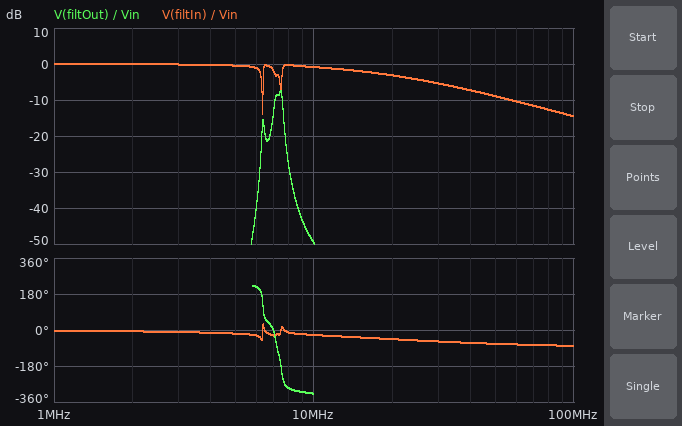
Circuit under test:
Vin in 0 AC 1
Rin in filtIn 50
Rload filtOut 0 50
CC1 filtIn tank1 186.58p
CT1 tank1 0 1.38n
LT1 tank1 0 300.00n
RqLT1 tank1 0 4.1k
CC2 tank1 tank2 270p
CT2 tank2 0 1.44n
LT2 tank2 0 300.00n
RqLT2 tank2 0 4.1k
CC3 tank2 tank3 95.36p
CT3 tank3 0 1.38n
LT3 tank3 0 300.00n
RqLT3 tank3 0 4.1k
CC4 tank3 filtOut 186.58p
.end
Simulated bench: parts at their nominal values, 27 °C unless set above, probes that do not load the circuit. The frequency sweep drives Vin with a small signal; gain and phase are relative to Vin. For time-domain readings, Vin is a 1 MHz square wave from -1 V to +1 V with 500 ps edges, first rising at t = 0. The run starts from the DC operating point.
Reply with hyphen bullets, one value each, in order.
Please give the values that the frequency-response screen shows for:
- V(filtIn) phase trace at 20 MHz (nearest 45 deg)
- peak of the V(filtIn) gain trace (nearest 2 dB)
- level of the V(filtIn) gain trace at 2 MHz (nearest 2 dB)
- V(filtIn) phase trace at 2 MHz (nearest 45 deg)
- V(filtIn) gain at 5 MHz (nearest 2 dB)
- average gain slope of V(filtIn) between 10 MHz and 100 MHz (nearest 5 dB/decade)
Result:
- -45 deg
- 0 dB
- 0 dB
- 0 deg
- 0 dB
- -15 dB/decade
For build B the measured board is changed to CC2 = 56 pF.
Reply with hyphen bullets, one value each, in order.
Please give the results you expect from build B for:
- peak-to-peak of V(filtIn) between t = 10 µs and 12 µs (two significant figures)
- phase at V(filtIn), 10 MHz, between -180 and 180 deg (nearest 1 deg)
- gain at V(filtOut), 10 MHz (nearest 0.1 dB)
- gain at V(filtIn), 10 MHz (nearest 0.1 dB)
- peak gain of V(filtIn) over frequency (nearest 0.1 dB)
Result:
- 2.2 V
- -24 deg
- -59.6 dB
- -0.8 dB
- 0 dB
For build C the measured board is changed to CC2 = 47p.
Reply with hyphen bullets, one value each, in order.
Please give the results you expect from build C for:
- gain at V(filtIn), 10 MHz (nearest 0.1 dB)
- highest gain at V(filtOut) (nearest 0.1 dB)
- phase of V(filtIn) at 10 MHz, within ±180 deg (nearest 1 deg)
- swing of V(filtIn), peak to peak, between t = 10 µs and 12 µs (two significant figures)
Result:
- -0.8 dB
- -8.2 dB
- -24 deg
- 2.2 V
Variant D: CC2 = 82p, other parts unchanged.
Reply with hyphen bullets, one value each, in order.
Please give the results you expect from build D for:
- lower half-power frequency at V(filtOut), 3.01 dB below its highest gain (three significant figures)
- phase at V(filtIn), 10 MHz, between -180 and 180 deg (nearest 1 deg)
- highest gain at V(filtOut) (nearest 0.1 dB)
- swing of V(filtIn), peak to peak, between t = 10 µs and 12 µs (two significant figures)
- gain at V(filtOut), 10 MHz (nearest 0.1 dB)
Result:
- 6.93 MHz
- -24 deg
- -7.0 dB
- 2.2 V
- -56.9 dB
